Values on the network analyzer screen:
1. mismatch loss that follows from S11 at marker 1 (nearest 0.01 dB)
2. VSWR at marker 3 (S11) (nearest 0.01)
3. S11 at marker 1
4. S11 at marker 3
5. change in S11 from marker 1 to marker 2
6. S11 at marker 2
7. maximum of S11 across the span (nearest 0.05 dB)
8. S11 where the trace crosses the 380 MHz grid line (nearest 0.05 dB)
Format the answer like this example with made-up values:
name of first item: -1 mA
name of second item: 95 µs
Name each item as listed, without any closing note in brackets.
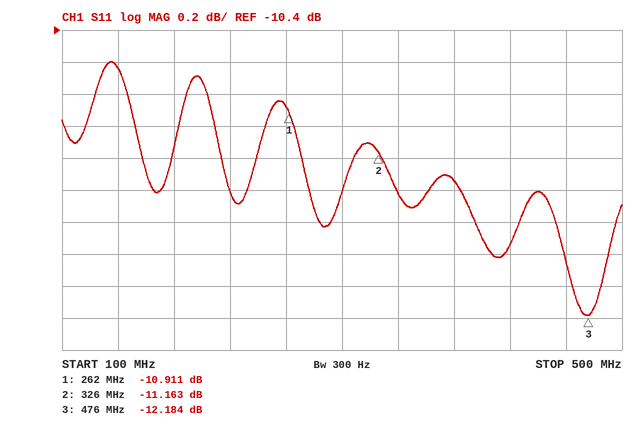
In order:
mismatch loss that follows from S11 at marker 1: 0.37 dB
VSWR at marker 3 (S11): 1.65
S11 at marker 1: -10.911 dB
S11 at marker 3: -12.184 dB
change in S11 from marker 1 to marker 2: -0.252 dB
S11 at marker 2: -11.163 dB
maximum of S11 across the span: -10.60 dB
S11 where the trace crosses the 380 MHz grid line: -11.35 dB
